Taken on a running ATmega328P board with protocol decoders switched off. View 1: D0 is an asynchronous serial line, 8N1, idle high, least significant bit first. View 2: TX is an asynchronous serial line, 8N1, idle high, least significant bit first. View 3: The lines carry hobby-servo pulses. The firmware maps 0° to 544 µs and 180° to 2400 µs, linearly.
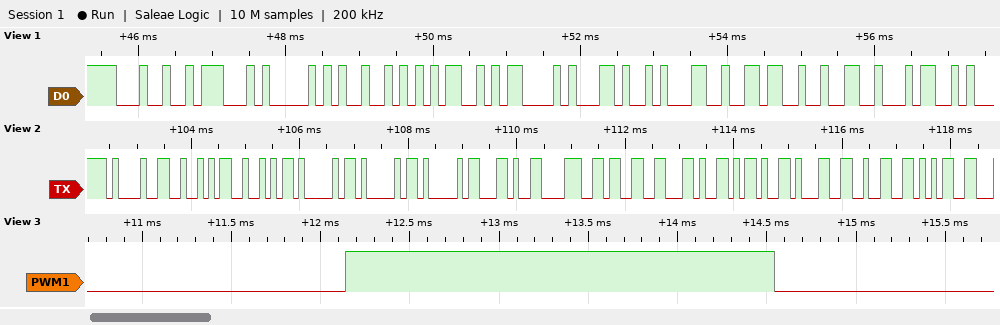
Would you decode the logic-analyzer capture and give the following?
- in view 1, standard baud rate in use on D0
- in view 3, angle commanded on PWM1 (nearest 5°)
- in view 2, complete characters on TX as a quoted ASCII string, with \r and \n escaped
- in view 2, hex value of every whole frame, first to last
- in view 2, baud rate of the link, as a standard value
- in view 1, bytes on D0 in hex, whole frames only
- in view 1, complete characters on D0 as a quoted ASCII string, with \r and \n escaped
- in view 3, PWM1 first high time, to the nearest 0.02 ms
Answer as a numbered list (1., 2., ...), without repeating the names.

1. 9600 baud
2. 180°
3. "!RRAAA,83,-125"
4. 21 52 52 41 41 41 2C 38 33 2C 2D 31 32 35
5. 9600 baud
6. 0x24 0x47 0x50 0x52 0x4D 0x43 0x2C 0x31 0x36 0x32 0x34
7. "$GPRMC,1624"
8. 2.40 ms
